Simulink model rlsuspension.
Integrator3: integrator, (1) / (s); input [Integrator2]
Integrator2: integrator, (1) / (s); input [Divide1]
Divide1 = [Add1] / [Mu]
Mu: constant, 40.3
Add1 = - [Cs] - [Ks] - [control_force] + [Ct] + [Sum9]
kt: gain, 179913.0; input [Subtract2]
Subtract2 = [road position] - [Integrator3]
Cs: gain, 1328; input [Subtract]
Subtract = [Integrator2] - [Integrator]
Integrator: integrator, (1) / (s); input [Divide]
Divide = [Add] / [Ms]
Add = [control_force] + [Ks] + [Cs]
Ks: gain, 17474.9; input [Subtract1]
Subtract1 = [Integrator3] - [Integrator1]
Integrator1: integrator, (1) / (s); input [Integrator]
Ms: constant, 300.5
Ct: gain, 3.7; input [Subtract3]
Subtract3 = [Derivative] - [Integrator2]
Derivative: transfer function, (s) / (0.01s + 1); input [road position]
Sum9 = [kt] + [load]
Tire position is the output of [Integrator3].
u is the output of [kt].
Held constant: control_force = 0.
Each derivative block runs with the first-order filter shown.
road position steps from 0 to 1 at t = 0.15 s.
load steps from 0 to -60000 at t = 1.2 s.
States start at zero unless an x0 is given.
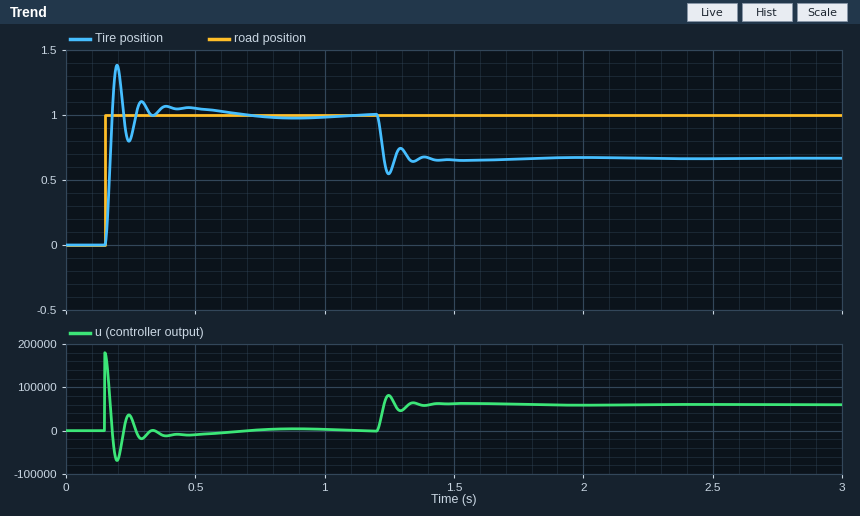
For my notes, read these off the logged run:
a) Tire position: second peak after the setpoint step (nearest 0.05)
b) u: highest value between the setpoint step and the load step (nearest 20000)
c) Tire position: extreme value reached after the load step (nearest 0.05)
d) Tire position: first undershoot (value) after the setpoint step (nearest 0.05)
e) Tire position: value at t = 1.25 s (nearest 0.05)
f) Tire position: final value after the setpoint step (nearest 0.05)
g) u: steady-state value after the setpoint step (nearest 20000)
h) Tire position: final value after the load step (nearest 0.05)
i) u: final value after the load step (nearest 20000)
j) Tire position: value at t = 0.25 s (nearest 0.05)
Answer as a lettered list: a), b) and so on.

a) 1.10
b) 180000
c) 0.55
d) 0.80
e) 0.55
f) 1.00
g) 0
h) 0.65
i) 60000
j) 0.80
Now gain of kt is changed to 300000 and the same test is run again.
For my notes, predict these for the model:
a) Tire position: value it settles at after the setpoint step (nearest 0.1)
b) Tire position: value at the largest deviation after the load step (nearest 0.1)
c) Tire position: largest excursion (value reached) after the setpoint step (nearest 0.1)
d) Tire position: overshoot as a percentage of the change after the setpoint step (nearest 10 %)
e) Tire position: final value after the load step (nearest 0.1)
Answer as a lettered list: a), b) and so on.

a) 1.0
b) 0.7
c) 1.5
d) 50 %
e) 0.8
